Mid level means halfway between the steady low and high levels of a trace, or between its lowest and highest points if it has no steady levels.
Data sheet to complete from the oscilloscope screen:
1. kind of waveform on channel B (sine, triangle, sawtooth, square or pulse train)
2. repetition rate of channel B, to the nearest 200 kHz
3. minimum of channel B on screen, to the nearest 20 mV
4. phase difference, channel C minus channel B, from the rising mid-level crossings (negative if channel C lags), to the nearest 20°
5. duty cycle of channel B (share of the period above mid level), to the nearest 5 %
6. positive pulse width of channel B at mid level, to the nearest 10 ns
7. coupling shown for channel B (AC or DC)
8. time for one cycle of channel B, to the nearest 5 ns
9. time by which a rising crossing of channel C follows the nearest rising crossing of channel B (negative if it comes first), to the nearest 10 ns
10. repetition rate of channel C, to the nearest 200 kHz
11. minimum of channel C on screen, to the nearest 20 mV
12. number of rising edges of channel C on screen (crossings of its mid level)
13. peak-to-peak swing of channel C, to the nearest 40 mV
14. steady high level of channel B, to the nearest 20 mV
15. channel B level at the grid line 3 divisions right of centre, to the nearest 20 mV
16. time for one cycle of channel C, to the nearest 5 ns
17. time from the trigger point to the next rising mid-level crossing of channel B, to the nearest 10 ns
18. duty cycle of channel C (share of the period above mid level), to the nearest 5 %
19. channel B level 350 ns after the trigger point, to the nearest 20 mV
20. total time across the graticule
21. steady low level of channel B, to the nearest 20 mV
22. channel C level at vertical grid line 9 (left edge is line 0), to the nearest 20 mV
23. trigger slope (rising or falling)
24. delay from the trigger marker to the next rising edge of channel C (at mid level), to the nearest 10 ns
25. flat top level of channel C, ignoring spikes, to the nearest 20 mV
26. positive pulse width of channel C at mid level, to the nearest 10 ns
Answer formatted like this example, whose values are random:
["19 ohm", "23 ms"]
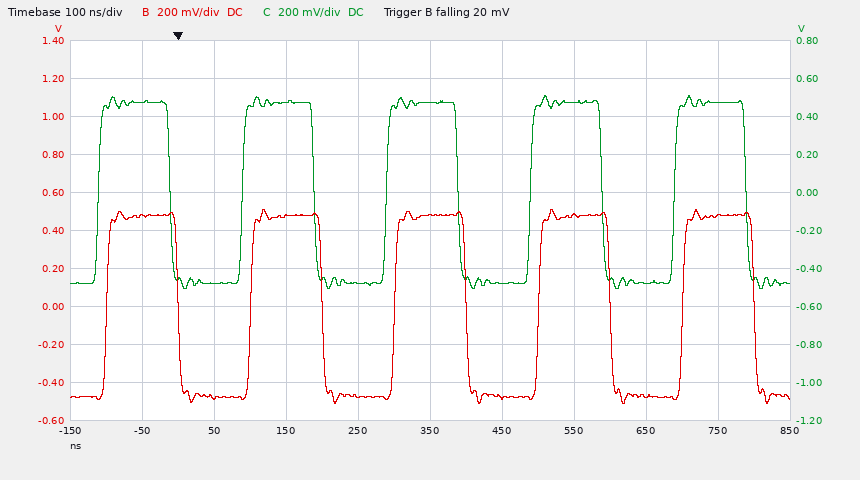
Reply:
["square", "5.0 MHz", "-520 mV", "+20°", "50 %", "100 ns", "DC", "200 ns", "-10 ns", "5.0 MHz", "-500 mV", "5", "1.00 V", "480 mV", "-480 mV", "200 ns", "100 ns", "50 %", "480 mV", "1 µs", "-480 mV", "480 mV", "falling", "90 ns", "480 mV", "100 ns"]
